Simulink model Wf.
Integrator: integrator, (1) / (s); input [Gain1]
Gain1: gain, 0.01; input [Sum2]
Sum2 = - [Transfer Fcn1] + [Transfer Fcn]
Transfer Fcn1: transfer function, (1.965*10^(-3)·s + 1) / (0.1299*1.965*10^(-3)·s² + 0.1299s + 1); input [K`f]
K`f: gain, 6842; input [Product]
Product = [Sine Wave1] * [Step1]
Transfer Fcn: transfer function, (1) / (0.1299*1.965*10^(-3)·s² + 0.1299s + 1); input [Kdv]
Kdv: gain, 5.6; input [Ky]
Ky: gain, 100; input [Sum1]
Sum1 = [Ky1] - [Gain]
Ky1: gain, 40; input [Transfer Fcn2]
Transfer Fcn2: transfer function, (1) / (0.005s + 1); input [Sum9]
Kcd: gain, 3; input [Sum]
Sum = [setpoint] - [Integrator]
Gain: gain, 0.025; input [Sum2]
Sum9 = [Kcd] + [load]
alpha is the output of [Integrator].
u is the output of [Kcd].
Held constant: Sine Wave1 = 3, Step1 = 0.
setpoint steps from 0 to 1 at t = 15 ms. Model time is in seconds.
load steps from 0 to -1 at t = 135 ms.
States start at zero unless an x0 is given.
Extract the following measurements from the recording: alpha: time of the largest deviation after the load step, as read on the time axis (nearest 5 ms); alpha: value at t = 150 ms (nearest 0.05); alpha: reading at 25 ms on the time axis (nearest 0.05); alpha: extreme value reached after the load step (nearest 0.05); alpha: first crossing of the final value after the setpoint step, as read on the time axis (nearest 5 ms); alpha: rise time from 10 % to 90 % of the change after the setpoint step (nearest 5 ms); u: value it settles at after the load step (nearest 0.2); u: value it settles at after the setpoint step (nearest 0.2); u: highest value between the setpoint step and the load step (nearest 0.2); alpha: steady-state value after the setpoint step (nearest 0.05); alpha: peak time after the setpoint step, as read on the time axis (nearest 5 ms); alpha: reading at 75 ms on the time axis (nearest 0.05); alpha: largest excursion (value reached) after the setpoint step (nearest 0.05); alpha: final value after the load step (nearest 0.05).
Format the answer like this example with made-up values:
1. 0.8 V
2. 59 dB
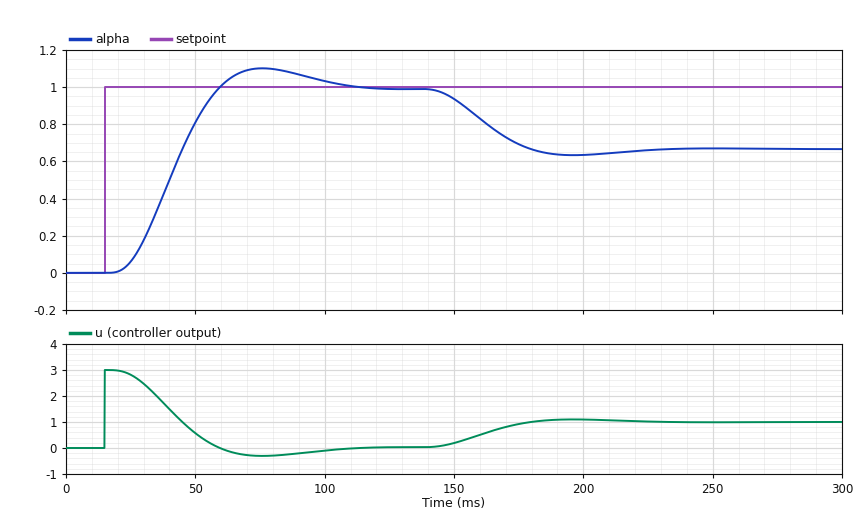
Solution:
1. 195 ms
2. 0.95
3. 0.05
4. 0.65
5. 60 ms
6. 25 ms
7. 1.0
8. 0.0
9. 3.0
10. 1.00
11. 75 ms
12. 1.10
13. 1.10
14. 0.65
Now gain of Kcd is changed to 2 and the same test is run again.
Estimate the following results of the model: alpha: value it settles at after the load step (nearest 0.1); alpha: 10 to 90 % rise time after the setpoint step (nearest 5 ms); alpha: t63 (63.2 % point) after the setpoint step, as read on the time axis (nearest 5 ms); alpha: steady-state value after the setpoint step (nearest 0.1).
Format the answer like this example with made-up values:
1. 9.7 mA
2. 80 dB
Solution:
1. 0.5
2. 45 ms
3. 55 ms
4. 1.0
